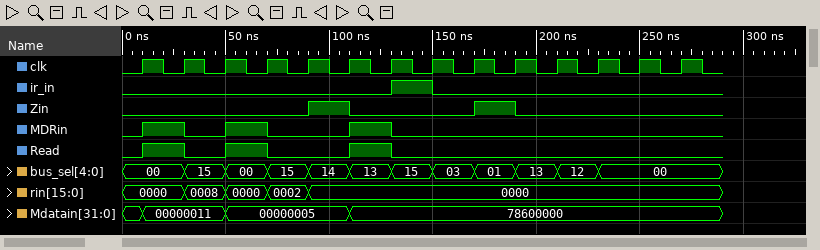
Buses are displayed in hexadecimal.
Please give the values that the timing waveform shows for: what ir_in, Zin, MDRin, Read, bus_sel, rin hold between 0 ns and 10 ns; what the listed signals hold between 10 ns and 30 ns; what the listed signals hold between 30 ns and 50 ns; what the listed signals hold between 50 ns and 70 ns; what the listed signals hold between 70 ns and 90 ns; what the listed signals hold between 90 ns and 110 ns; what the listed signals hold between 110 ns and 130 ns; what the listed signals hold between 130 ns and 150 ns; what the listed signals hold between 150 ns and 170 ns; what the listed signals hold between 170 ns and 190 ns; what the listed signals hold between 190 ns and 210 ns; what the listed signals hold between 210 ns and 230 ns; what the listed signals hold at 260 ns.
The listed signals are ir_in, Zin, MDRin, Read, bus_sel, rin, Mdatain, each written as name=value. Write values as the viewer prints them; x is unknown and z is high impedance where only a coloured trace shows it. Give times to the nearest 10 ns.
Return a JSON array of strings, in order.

["ir_in=0, Zin=0, MDRin=0, Read=0, bus_sel=00, rin=0000", "ir_in=0, Zin=0, MDRin=1, Read=1, bus_sel=00, rin=0000, Mdatain=00000011", "ir_in=0, Zin=0, MDRin=0, Read=0, bus_sel=15, rin=0008, Mdatain=00000011", "ir_in=0, Zin=0, MDRin=1, Read=1, bus_sel=00, rin=0000, Mdatain=00000005", "ir_in=0, Zin=0, MDRin=0, Read=0, bus_sel=15, rin=0002, Mdatain=00000005", "ir_in=0, Zin=1, MDRin=0, Read=0, bus_sel=14, rin=0000, Mdatain=00000005", "ir_in=0, Zin=0, MDRin=1, Read=1, bus_sel=13, rin=0000, Mdatain=78600000", "ir_in=1, Zin=0, MDRin=0, Read=0, bus_sel=15, rin=0000, Mdatain=78600000", "ir_in=0, Zin=0, MDRin=0, Read=0, bus_sel=03, rin=0000, Mdatain=78600000", "ir_in=0, Zin=1, MDRin=0, Read=0, bus_sel=01, rin=0000, Mdatain=78600000", "ir_in=0, Zin=0, MDRin=0, Read=0, bus_sel=13, rin=0000, Mdatain=78600000", "ir_in=0, Zin=0, MDRin=0, Read=0, bus_sel=12, rin=0000, Mdatain=78600000", "ir_in=0, Zin=0, MDRin=0, Read=0, bus_sel=00, rin=0000, Mdatain=78600000"]
